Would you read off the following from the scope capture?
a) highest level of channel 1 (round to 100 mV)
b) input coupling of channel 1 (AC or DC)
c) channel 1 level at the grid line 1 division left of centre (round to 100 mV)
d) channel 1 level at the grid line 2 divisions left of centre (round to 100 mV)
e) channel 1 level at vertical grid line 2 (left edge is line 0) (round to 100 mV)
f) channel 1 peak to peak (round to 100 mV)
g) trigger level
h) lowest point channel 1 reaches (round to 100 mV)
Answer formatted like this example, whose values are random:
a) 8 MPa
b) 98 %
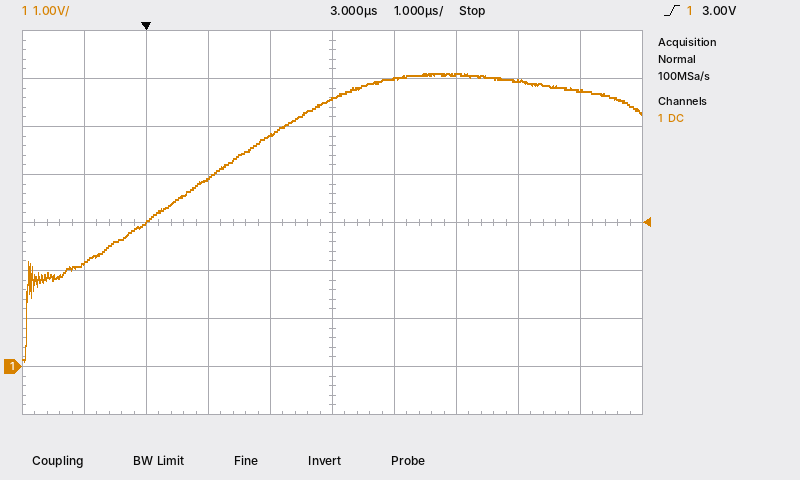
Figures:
a) 6.1 V
b) DC
c) 4.8 V
d) 3.9 V
e) 3.0 V
f) 6.0 V
g) 3.00 V
h) 100 mV
